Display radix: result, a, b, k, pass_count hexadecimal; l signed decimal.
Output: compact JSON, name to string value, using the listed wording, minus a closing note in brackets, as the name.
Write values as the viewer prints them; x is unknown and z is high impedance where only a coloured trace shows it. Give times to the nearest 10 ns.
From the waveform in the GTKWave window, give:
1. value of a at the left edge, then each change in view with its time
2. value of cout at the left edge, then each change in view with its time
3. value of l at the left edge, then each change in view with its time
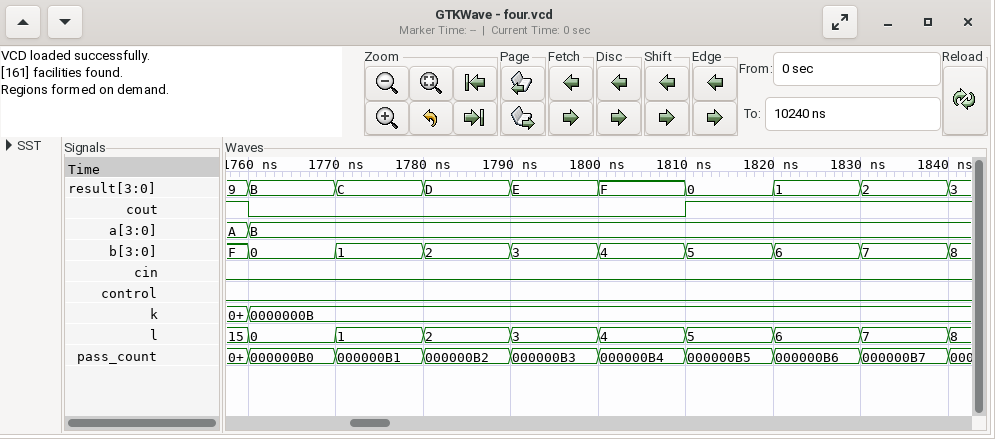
{"value of a at the left edge, then each change in view with its time": "A, B at 1760 ns", "value of cout at the left edge, then each change in view with its time": "1, 0 at 1760 ns, 1 at 1810 ns", "value of l at the left edge, then each change in view with its time": "15, 0 at 1760 ns, 1 at 1770 ns, 2 at 1780 ns, 3 at 1790 ns, 4 at 1800 ns, 5 at 1810 ns, 6 at 1820 ns, 7 at 1830 ns, 8 at 1840 ns"}
